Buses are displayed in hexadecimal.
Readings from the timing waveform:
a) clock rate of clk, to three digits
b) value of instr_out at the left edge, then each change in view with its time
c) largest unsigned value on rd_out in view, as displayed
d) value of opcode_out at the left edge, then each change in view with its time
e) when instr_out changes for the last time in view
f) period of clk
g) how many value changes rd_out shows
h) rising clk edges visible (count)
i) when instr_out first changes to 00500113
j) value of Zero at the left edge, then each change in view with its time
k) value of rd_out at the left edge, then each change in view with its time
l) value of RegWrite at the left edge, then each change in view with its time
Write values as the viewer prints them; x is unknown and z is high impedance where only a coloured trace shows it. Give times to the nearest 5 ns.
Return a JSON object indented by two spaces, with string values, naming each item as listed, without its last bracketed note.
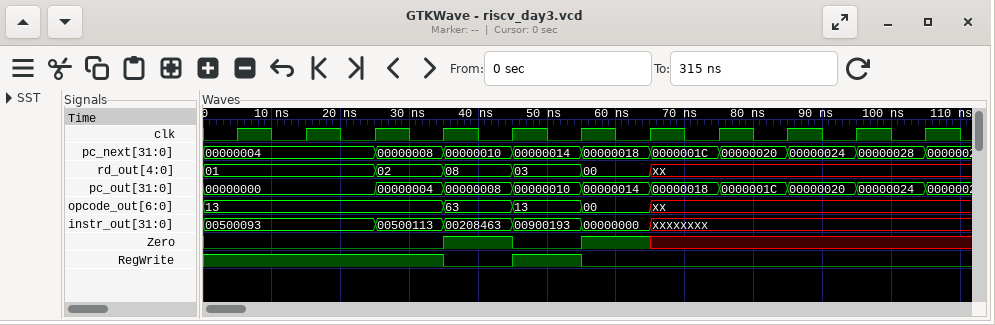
{
  "clock rate of clk, to three digits": "100 MHz",
  "value of instr_out at the left edge, then each change in view with its time": "00500093, 00500113 at 25 ns, 00208463 at 35 ns, 00900193 at 45 ns, 00000000 at 55 ns, xxxxxxxx at 65 ns",
  "largest unsigned value on rd_out in view, as displayed": "08",
  "value of opcode_out at the left edge, then each change in view with its time": "13, 63 at 35 ns, 13 at 45 ns, 00 at 55 ns, xx at 65 ns",
  "when instr_out changes for the last time in view": "65 ns",
  "period of clk": "10 ns",
  "how many value changes rd_out shows": "5",
  "rising clk edges visible": "11",
  "when instr_out first changes to 00500113": "25 ns",
  "value of Zero at the left edge, then each change in view with its time": "0, 1 at 35 ns, 0 at 45 ns, 1 at 55 ns, x at 65 ns",
  "value of rd_out at the left edge, then each change in view with its time": "01, 02 at 25 ns, 08 at 35 ns, 03 at 45 ns, 00 at 55 ns, xx at 65 ns",
  "value of RegWrite at the left edge, then each change in view with its time": "1, 0 at 35 ns, 1 at 45 ns, 0 at 55 ns"
}
